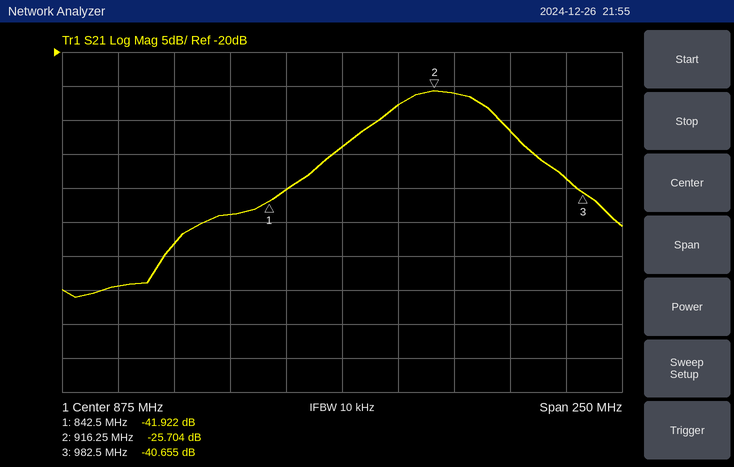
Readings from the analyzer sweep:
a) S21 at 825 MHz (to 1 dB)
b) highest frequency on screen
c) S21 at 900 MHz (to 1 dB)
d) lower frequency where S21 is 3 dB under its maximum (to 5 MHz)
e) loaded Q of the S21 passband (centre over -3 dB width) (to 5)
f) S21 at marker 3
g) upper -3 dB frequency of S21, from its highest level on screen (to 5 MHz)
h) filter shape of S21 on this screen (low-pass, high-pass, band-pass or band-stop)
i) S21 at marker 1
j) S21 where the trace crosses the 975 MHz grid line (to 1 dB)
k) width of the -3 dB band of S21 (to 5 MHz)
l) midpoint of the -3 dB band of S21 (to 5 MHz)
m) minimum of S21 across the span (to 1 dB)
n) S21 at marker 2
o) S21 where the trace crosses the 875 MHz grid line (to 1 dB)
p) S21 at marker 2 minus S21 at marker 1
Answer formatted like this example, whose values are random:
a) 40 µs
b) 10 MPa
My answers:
a) -44 dB
b) 1 GHz
c) -28 dB
d) 895 MHz
e) 20
f) -40.655 dB
g) 940 MHz
h) band-pass
i) -41.922 dB
j) -39 dB
k) 45 MHz
l) 920 MHz
m) -56 dB
n) -25.704 dB
o) -34 dB
p) 16.218 dB
